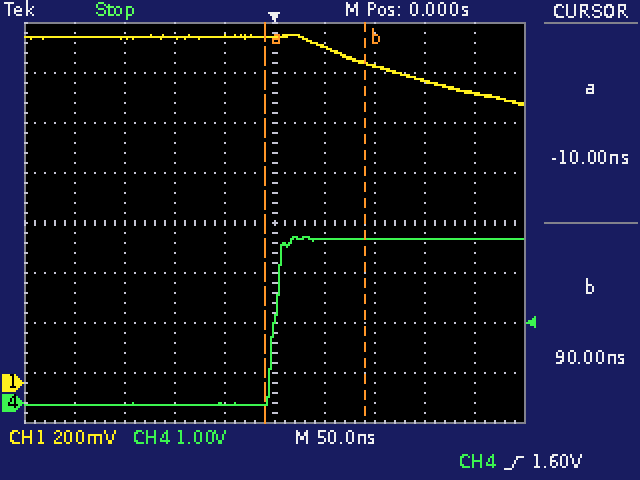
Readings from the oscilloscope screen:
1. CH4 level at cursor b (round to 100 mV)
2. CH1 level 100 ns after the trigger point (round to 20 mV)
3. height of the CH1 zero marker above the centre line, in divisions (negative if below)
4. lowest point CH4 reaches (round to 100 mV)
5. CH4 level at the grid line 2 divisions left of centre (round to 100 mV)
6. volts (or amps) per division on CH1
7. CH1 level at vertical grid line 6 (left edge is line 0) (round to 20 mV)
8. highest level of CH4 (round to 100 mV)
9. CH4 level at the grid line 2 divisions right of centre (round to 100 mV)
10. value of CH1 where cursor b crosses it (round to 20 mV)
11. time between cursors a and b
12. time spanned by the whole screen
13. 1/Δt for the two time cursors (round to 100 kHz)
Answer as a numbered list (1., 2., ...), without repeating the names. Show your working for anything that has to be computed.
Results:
1. 3.3 V
2. 1.26 V
3. -3.2 div
4. 0.0 V
5. 0.0 V
6. 200 mV
7. 1.34 V
8. 3.3 V
9. 3.3 V
10. 1.28 V
11. 90 ns − (-10 ns) = 100 ns
12. 500 ns
13. 1 / 100 ns ≈ 10.0 MHz
